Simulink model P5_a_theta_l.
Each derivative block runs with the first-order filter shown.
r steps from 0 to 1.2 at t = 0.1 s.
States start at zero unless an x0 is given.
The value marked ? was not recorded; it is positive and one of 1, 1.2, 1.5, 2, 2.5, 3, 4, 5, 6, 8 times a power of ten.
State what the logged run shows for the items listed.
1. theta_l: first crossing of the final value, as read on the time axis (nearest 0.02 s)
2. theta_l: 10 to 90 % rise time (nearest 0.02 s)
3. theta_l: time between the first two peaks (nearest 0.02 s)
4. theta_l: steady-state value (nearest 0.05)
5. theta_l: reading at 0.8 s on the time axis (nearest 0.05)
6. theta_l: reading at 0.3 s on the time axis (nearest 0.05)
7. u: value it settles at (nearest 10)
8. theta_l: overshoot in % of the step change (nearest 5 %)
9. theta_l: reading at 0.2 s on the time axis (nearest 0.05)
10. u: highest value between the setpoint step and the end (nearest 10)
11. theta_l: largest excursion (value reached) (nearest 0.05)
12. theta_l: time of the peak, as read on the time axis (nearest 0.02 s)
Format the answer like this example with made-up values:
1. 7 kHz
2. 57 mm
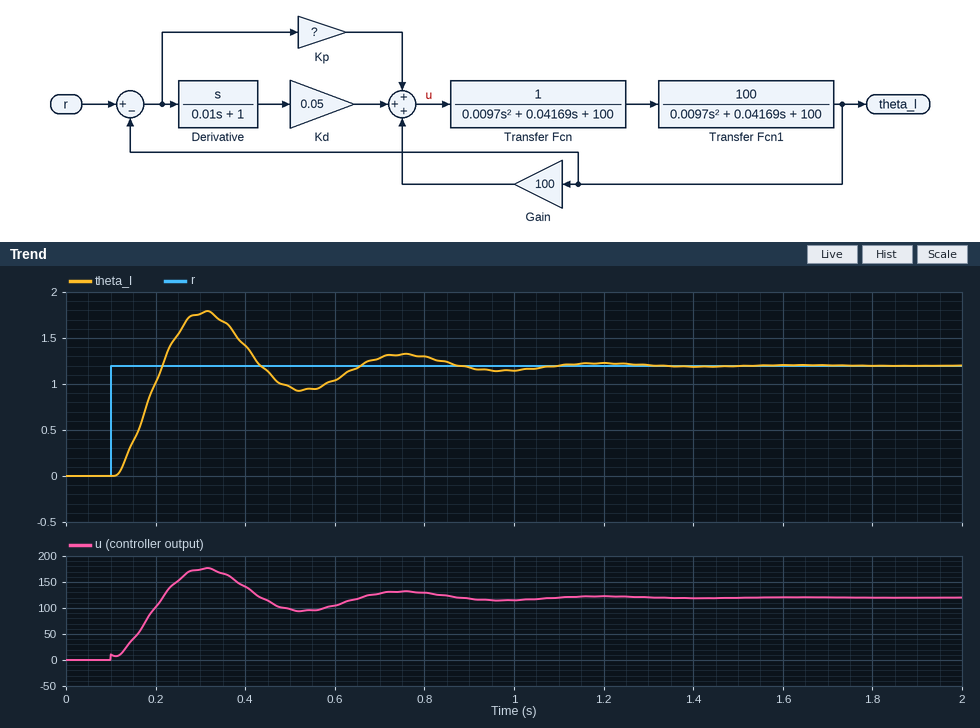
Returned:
1. 0.22 s
2. 0.08 s
3. 0.44 s
4. 1.20
5. 1.30
6. 1.75
7. 120
8. 50 %
9. 1.00
10. 180
11. 1.80
12. 0.32 s
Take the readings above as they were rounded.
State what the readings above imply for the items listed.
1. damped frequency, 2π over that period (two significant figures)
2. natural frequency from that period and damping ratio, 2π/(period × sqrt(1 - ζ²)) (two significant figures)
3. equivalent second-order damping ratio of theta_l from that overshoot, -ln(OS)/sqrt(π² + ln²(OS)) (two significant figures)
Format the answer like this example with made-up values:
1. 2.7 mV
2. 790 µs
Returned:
1. 14 rad/s
2. 15 rad/s
3. 0.22
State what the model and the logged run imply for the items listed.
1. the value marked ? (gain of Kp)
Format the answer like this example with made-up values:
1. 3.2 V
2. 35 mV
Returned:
1. 4
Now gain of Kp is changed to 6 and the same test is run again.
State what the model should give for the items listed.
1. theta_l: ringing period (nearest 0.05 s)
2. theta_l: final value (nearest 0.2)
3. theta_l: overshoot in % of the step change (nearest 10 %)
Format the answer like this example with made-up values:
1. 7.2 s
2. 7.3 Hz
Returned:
1. 0.35 s
2. 1.2
3. 60 %
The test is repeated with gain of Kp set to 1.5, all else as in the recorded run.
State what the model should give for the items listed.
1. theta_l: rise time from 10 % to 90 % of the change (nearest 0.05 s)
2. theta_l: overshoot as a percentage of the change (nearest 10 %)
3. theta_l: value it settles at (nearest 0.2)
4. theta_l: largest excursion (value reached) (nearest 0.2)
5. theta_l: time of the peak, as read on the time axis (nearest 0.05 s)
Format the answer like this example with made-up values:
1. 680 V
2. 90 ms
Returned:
1. 0.15 s
2. 30 %
3. 1.2
4. 1.6
5. 0.45 s
